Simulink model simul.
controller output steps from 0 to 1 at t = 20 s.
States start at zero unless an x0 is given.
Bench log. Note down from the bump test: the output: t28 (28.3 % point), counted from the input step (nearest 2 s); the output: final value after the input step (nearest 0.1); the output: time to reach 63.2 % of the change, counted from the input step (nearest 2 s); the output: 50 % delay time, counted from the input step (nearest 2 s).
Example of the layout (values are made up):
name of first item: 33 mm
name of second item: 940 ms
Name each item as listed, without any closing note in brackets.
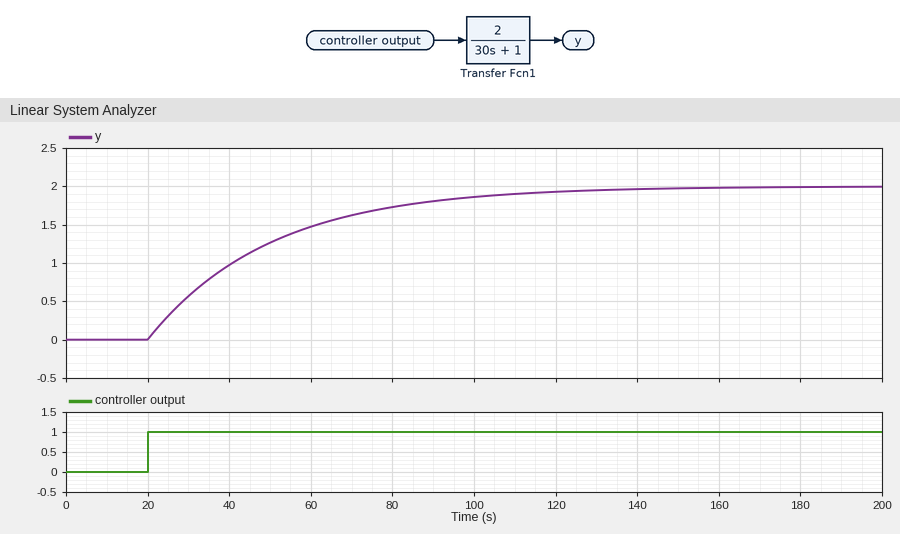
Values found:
the output: t28 (28.3 % point), counted from the input step: 10 s
the output: final value after the input step: 2.0
the output: time to reach 63.2 % of the change, counted from the input step: 30 s
the output: 50 % delay time, counted from the input step: 20 s
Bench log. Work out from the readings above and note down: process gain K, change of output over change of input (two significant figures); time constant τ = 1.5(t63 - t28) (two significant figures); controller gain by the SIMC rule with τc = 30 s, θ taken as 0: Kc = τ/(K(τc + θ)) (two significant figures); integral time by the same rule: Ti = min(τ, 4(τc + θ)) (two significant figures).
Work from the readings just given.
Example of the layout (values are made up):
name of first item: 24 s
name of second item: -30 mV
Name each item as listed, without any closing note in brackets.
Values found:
process gain K, change of output over change of input: 2.0
time constant τ = 1.5(t63 - t28): 30 s
controller gain by the SIMC rule with τc = 30 s, θ taken as 0: Kc = τ/(K(τc + θ)): 0.50
integral time by the same rule: Ti = min(τ, 4(τc + θ)): 30 s
